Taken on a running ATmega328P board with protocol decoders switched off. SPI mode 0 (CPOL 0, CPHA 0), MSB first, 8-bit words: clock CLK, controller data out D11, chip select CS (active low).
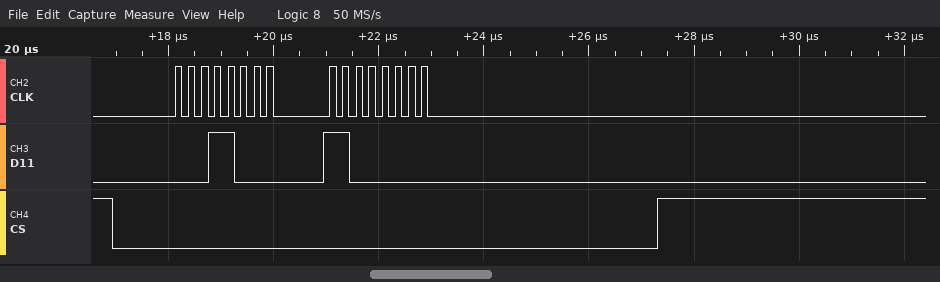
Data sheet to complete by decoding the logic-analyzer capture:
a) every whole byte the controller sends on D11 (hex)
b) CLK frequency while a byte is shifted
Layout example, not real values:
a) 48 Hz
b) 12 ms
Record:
a) 18 C0
b) 4 MHz
